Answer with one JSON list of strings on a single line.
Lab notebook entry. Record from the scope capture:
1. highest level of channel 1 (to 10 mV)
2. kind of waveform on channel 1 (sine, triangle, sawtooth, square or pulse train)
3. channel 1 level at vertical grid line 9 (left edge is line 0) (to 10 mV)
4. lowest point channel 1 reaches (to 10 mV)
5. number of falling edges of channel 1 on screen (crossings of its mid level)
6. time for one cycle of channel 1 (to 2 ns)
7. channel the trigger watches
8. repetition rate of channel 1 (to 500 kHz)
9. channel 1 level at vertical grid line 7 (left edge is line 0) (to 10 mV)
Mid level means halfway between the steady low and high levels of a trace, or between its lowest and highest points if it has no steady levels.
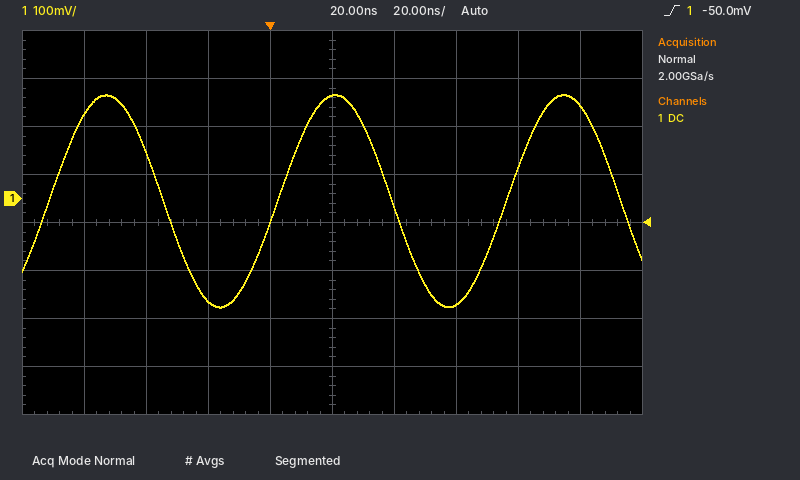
["220 mV", "sine", "190 mV", "-230 mV", "3", "74 ns", "channel 1", "13.5 MHz", "-220 mV"]
